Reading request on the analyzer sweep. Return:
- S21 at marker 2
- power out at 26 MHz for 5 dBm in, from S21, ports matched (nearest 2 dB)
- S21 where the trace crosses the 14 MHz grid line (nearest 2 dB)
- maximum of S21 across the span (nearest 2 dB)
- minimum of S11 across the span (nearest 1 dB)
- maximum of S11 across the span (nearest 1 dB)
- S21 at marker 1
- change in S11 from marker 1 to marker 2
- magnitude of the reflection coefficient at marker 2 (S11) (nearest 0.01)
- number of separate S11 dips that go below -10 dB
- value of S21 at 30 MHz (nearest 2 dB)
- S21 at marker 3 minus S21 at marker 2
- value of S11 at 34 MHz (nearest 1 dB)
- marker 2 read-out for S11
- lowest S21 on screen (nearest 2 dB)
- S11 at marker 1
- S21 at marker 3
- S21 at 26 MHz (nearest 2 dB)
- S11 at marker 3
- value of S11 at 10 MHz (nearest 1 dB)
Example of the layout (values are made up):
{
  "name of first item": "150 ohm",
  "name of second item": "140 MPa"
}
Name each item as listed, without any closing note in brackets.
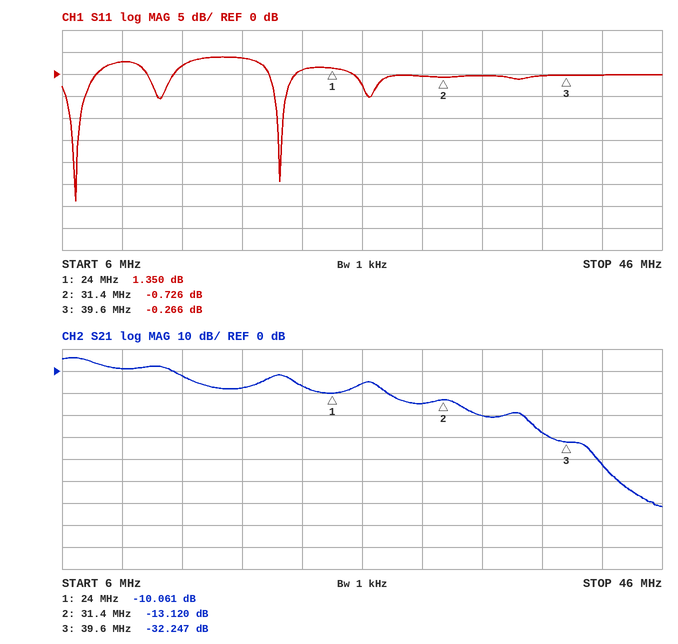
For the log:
{
  "S21 at marker 2": "-13.120 dB",
  "power out at 26 MHz for 5 dBm in, from S21, ports matched": "0 dBm",
  "S21 where the trace crosses the 14 MHz grid line": "-2 dB",
  "maximum of S21 across the span": "6 dB",
  "minimum of S11 across the span": "-29 dB",
  "maximum of S11 across the span": "4 dB",
  "S21 at marker 1": "-10.061 dB",
  "change in S11 from marker 1 to marker 2": "-2.076 dB",
  "magnitude of the reflection coefficient at marker 2 (S11)": "0.92",
  "number of separate S11 dips that go below -10 dB": "2",
  "value of S21 at 30 MHz": "-14 dB",
  "S21 at marker 3 minus S21 at marker 2": "-19.127 dB",
  "value of S11 at 34 MHz": "0 dB",
  "marker 2 read-out for S11": "-0.726 dB",
  "lowest S21 on screen": "-62 dB",
  "S11 at marker 1": "1.350 dB",
  "S21 at marker 3": "-32.247 dB",
  "S21 at 26 MHz": "-6 dB",
  "S11 at marker 3": "-0.266 dB",
  "value of S11 at 10 MHz": "3 dB"
}
